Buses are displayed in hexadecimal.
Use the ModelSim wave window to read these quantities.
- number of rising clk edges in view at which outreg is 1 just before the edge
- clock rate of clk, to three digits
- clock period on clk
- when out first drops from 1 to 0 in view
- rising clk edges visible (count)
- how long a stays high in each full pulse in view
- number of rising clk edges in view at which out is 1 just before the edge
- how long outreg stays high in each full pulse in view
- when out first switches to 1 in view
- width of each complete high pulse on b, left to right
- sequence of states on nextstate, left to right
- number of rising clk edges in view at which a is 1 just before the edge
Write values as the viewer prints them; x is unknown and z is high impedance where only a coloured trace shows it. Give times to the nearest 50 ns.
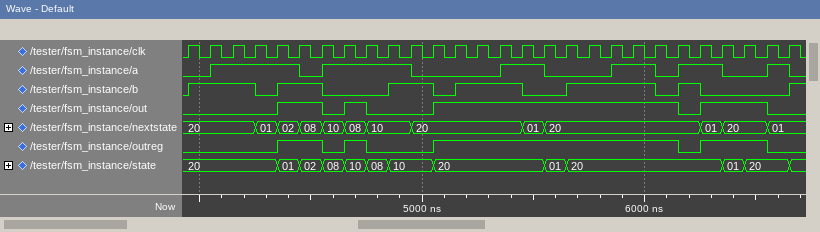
17
10.0 MHz
100 ns
4550 ns
28
400 ns, 400 ns, 200 ns, 200 ns, 200 ns, 100 ns
17
200 ns, 100 ns, 1100 ns, 300 ns
4350 ns
300 ns, 200 ns, 200 ns, 300 ns, 400 ns, 100 ns
20, 01, 02, 08, 10, 08, 10, 20, 01, 20, 01, 20, 01
15
